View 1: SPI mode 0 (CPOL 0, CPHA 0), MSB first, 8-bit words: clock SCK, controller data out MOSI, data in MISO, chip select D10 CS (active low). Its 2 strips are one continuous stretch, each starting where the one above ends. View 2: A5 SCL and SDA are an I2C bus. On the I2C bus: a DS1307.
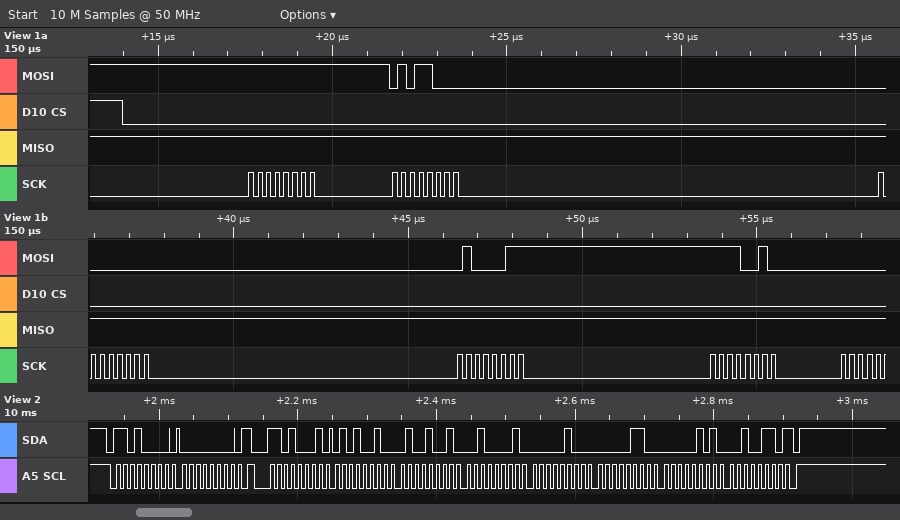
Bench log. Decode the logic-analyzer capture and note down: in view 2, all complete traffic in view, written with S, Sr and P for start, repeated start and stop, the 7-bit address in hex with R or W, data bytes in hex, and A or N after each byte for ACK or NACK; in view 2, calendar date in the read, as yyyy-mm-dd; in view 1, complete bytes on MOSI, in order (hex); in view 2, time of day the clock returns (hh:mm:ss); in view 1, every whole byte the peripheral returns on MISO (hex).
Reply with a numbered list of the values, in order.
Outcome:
1. S 68W A 00 A Sr 68R A 52 A 49 A 21 A 04 A 06 A 05 A 26 N P
2. 2026-05-06
3. FF 58 00 43 F2
4. 21:49:52
5. FF FF FF FF FF
